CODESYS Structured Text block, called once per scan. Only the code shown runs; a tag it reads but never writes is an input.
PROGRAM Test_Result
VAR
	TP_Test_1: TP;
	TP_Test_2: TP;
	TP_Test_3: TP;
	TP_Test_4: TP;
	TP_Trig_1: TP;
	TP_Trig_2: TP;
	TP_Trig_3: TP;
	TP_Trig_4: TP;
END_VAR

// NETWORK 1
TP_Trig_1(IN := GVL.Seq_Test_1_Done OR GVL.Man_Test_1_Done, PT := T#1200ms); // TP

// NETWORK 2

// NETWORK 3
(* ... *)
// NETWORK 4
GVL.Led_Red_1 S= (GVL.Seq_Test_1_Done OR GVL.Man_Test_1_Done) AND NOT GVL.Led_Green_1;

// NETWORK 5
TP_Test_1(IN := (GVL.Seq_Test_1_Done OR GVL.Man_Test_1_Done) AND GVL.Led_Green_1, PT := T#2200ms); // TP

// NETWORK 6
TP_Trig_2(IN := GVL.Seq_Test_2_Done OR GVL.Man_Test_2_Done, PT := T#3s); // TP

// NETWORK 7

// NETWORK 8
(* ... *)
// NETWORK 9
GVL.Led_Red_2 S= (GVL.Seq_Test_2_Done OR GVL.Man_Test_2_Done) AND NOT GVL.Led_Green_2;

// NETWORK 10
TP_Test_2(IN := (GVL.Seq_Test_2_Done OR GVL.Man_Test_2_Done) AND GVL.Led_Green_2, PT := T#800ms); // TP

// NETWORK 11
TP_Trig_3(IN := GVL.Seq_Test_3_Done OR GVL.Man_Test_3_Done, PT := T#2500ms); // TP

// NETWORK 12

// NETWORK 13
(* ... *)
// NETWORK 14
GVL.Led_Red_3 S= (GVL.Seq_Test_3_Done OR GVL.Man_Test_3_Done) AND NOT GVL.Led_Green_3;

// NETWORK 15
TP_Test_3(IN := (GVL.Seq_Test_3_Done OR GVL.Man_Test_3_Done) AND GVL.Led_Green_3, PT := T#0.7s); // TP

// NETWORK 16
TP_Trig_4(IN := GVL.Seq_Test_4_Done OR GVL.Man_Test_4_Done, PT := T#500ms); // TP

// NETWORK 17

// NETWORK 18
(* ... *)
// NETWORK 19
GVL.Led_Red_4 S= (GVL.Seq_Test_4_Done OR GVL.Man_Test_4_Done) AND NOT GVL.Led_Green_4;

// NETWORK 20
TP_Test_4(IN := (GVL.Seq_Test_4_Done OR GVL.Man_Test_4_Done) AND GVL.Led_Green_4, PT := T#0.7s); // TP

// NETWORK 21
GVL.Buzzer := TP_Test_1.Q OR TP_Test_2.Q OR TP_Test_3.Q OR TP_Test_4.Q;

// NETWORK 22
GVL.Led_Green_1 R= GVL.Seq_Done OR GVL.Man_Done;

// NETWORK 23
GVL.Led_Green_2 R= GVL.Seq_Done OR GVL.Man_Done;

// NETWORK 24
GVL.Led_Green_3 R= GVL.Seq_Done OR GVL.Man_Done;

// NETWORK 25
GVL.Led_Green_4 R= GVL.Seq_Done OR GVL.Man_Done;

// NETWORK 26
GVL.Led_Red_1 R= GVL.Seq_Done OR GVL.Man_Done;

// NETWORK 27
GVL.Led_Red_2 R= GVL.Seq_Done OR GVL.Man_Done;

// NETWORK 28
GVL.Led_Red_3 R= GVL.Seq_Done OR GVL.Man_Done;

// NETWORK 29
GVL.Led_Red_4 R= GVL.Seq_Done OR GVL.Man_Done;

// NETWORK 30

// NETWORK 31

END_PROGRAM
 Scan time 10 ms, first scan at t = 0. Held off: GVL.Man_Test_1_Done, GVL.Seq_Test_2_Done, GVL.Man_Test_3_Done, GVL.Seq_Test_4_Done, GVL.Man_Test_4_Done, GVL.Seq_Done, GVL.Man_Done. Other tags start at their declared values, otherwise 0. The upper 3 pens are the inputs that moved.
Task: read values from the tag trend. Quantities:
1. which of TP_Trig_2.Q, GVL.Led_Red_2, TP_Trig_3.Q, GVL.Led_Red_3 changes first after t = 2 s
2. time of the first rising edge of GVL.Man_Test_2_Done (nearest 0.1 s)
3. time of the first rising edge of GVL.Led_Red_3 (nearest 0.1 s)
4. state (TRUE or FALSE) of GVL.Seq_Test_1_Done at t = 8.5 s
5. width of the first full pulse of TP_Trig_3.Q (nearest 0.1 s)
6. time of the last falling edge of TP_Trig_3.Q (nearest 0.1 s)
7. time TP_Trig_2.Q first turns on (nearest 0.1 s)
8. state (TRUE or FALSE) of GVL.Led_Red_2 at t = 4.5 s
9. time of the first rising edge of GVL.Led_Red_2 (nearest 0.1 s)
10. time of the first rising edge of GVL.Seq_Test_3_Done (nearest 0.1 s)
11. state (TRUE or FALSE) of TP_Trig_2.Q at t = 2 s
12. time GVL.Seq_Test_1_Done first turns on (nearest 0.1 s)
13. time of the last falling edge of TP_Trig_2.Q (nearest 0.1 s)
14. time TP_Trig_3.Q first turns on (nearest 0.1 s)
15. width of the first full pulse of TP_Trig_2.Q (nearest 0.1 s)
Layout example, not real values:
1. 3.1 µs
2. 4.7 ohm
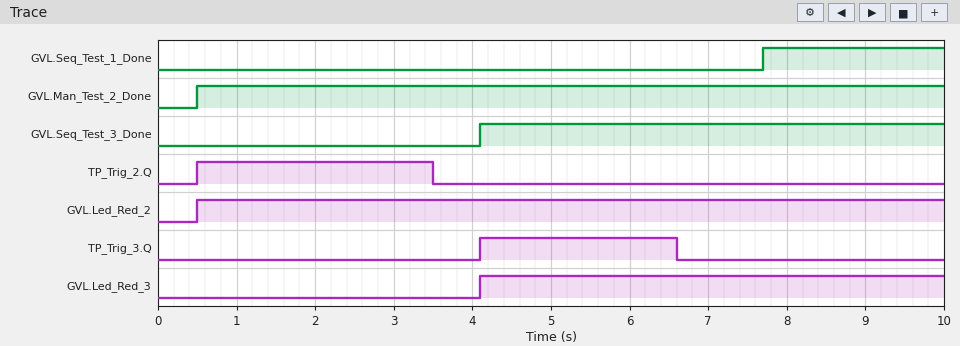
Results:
1. TP_Trig_2.Q
2. 0.5 s
3. 4.1 s
4. TRUE
5. 2.5 s
6. 6.6 s
7. 0.5 s
8. TRUE
9. 0.5 s
10. 4.1 s
11. TRUE
12. 7.7 s
13. 3.5 s
14. 4.1 s
15. 3.0 s
